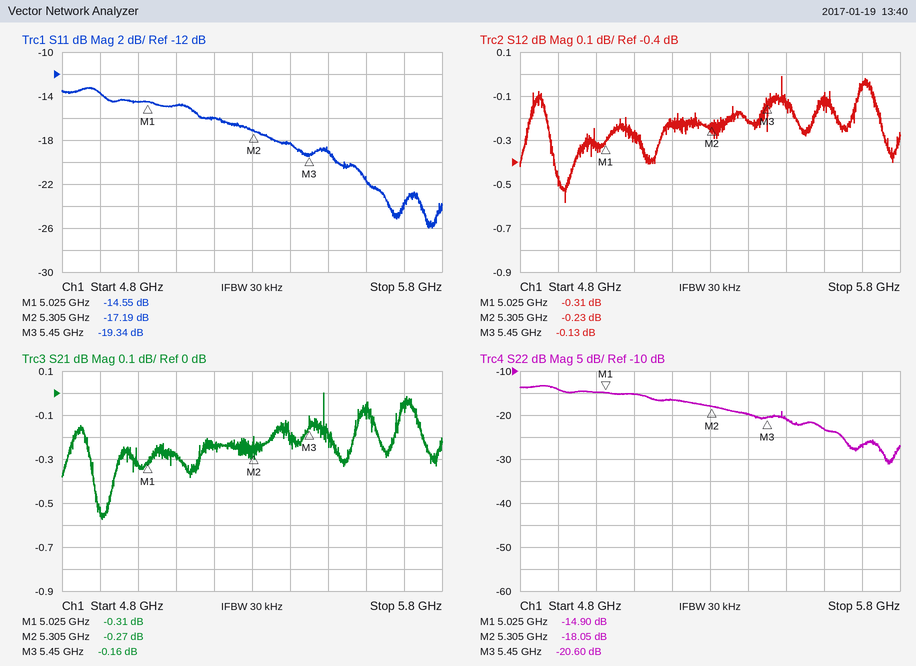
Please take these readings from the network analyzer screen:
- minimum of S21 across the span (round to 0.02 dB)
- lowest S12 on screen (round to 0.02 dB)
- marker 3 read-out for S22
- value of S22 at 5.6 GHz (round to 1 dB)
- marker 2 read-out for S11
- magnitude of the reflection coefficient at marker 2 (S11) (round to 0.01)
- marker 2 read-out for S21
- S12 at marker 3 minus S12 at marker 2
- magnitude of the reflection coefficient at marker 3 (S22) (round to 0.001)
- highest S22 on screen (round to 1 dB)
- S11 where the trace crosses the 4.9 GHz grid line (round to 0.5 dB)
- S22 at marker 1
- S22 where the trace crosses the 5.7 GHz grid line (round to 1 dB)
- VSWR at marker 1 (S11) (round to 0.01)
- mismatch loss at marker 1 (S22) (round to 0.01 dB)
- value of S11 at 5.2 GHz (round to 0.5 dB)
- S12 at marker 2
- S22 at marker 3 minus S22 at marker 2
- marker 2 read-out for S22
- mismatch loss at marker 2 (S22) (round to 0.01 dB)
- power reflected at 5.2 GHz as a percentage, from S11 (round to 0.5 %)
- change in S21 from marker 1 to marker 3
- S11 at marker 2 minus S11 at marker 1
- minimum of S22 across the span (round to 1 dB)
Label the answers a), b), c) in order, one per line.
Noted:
a) -0.58 dB
b) -0.58 dB
c) -20.60 dB
d) -23 dB
e) -17.19 dB
f) 0.14
g) -0.27 dB
h) 0.10 dB
i) 0.093
j) -13 dB
k) -13.5 dB
l) -14.90 dB
m) -27 dB
n) 1.46
o) 0.14 dB
p) -16.0 dB
q) -0.23 dB
r) -2.55 dB
s) -18.05 dB
t) 0.07 dB
u) 2.5 %
v) 0.15 dB
w) -2.64 dB
x) -31 dB
